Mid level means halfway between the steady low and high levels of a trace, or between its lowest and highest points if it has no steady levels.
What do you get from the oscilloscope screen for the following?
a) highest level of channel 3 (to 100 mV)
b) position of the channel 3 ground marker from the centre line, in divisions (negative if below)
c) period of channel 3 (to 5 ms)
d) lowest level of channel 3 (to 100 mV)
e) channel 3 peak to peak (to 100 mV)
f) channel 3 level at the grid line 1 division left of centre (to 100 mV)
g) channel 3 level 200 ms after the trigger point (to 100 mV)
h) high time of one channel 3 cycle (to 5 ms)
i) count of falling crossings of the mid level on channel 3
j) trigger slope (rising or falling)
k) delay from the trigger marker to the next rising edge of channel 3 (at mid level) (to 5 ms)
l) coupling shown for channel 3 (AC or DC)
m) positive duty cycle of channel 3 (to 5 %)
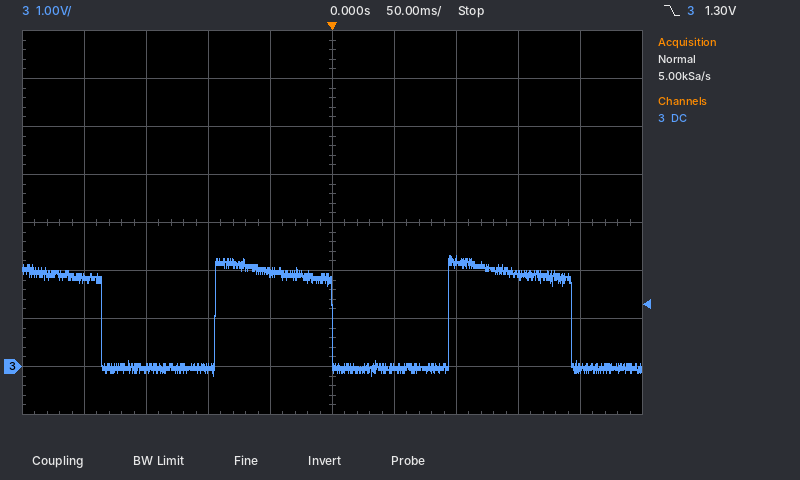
2.3 V
-3.0 div
190 ms
-200 mV
2.5 V
2.0 V
0.0 V
95 ms
3
falling
95 ms
DC
50 %
